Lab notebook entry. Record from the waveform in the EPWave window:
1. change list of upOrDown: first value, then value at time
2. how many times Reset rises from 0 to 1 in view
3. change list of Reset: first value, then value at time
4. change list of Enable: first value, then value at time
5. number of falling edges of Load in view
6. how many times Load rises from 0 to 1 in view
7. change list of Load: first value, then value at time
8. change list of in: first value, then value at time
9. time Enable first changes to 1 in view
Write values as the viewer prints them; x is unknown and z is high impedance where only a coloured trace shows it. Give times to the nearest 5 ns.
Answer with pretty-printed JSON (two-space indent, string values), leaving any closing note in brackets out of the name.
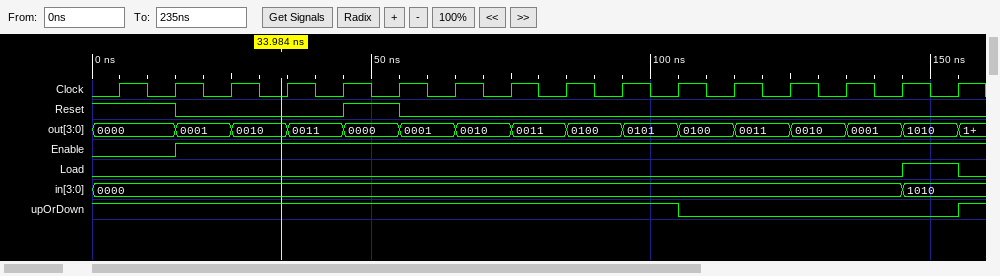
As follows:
{
  "change list of upOrDown: first value, then value at time": "1, 0 at 105 ns, 1 at 155 ns",
  "how many times Reset rises from 0 to 1 in view": "1",
  "change list of Reset: first value, then value at time": "1, 0 at 15 ns, 1 at 45 ns, 0 at 55 ns",
  "change list of Enable: first value, then value at time": "0, 1 at 15 ns",
  "number of falling edges of Load in view": "1",
  "how many times Load rises from 0 to 1 in view": "1",
  "change list of Load: first value, then value at time": "0, 1 at 145 ns, 0 at 155 ns",
  "change list of in: first value, then value at time": "0000, 1010 at 145 ns",
  "time Enable first changes to 1 in view": "15 ns"
}
